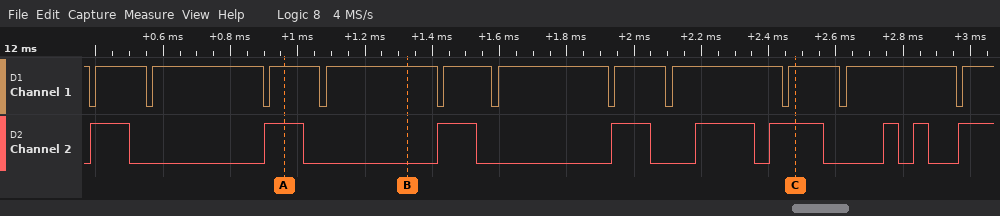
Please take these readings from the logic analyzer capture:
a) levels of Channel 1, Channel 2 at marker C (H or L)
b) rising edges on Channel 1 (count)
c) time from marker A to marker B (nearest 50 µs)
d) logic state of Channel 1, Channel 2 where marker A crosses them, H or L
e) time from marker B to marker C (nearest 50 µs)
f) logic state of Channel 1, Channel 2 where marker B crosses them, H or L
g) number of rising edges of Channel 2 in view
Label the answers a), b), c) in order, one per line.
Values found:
a) Channel 1=H, Channel 2=H
b) 11
c) 350 µs
d) Channel 1=H, Channel 2=H
e) 1150 µs
f) Channel 1=H, Channel 2=L
g) 9
